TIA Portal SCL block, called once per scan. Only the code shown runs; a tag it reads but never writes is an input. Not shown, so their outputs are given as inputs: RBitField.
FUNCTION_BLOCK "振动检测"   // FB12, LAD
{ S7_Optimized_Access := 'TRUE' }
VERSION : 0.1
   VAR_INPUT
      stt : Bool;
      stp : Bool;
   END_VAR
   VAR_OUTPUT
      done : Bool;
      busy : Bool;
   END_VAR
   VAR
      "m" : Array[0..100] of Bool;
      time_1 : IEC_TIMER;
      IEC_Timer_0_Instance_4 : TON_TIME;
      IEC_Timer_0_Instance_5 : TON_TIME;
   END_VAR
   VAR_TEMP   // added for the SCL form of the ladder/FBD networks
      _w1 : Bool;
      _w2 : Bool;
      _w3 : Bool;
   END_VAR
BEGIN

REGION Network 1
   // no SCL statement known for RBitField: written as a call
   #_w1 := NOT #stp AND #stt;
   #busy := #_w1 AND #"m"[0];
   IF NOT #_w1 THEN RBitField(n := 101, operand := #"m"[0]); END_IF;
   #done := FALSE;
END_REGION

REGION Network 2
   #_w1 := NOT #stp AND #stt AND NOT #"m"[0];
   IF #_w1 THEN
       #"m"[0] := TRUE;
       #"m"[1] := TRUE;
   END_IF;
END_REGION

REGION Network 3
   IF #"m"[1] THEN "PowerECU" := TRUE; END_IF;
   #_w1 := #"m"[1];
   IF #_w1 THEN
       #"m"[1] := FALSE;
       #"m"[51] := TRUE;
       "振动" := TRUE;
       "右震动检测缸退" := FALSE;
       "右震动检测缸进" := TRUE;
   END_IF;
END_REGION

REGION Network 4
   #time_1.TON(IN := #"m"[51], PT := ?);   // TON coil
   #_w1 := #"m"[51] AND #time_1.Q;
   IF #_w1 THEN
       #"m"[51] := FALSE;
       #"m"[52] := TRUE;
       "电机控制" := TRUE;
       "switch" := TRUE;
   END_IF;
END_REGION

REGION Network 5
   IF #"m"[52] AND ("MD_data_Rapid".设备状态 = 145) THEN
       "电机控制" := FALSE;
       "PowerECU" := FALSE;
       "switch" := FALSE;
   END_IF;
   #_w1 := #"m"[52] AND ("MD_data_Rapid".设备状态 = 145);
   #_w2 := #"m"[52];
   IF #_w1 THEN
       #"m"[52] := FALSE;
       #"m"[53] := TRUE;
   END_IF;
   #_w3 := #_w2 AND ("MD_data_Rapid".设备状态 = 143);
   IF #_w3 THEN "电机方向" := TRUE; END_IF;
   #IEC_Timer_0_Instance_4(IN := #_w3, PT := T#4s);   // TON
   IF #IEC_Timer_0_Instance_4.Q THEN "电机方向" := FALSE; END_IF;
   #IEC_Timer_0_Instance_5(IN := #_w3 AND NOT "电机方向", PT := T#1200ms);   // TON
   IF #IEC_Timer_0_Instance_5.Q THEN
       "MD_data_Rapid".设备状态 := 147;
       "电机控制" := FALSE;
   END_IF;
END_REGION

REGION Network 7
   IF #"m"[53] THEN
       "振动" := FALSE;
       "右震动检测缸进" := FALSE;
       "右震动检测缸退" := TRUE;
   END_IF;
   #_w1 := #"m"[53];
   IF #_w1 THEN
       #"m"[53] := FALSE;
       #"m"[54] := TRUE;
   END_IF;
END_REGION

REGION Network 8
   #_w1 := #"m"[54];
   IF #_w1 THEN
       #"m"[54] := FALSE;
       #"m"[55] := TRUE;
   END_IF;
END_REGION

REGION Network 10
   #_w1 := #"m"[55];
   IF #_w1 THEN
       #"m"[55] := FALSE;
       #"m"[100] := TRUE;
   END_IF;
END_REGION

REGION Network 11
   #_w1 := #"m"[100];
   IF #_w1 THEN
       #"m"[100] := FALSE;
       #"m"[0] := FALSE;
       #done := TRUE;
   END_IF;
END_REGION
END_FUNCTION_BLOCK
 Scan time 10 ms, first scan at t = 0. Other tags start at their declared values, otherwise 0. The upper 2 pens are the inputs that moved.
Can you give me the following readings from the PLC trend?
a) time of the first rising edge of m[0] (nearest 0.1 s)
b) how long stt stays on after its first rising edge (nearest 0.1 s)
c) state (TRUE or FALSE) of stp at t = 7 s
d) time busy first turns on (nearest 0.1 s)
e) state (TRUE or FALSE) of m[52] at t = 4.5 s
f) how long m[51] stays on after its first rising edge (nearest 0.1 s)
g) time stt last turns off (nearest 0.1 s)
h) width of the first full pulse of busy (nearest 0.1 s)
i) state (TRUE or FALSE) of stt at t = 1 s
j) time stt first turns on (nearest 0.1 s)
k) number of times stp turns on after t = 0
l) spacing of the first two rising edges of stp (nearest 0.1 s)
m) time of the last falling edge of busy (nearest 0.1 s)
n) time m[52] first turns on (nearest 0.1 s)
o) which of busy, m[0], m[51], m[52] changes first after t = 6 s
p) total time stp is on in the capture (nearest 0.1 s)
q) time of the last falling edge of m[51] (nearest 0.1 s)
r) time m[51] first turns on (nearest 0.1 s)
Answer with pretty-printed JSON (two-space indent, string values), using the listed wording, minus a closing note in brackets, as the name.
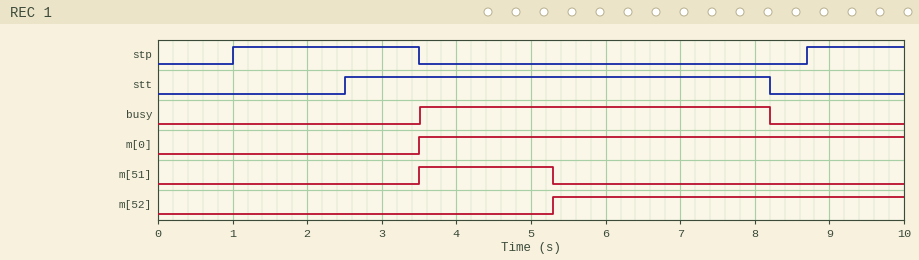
{
  "time of the first rising edge of m[0]": "3.5 s",
  "how long stt stays on after its first rising edge": "5.7 s",
  "state (TRUE or FALSE) of stp at t = 7 s": "FALSE",
  "time busy first turns on": "3.5 s",
  "state (TRUE or FALSE) of m[52] at t = 4.5 s": "FALSE",
  "how long m[51] stays on after its first rising edge": "1.8 s",
  "time stt last turns off": "8.2 s",
  "width of the first full pulse of busy": "4.7 s",
  "state (TRUE or FALSE) of stt at t = 1 s": "FALSE",
  "time stt first turns on": "2.5 s",
  "number of times stp turns on after t = 0": "2",
  "spacing of the first two rising edges of stp": "7.7 s",
  "time of the last falling edge of busy": "8.2 s",
  "time m[52] first turns on": "5.3 s",
  "which of busy, m[0], m[51], m[52] changes first after t = 6 s": "busy",
  "total time stp is on in the capture": "3.8 s",
  "time of the last falling edge of m[51]": "5.3 s",
  "time m[51] first turns on": "3.5 s"
}
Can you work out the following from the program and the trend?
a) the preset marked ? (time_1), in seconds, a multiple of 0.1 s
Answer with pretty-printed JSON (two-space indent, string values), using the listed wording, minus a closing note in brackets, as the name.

{
  "the preset marked ? (time_1), in seconds, a multiple of 0.1 s": "1.8 s"
}
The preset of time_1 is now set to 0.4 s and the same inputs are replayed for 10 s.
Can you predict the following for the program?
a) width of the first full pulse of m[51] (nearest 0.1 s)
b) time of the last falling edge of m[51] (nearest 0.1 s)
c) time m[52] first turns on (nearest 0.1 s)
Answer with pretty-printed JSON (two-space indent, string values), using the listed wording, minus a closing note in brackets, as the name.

{
  "width of the first full pulse of m[51]": "0.4 s",
  "time of the last falling edge of m[51]": "3.9 s",
  "time m[52] first turns on": "3.9 s"
}
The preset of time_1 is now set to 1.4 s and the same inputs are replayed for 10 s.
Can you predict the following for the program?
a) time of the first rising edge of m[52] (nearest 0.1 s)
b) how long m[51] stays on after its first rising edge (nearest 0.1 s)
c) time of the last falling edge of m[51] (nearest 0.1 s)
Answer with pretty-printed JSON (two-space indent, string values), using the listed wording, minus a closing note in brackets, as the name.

{
  "time of the first rising edge of m[52]": "4.9 s",
  "how long m[51] stays on after its first rising edge": "1.4 s",
  "time of the last falling edge of m[51]": "4.9 s"
}
